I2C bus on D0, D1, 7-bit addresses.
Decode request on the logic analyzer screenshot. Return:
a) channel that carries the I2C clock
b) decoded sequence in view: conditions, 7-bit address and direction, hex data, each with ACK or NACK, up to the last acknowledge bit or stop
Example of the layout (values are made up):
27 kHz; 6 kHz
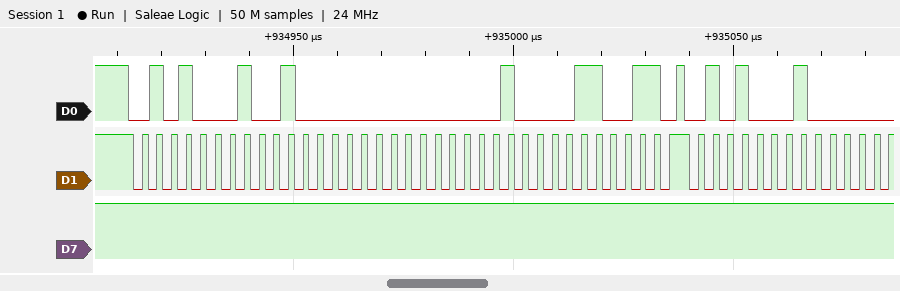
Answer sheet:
D1; start, address 28 read ACK, 40 ACK, 01 ACK, 19 NACK, stop, start, address 28 read ACK
